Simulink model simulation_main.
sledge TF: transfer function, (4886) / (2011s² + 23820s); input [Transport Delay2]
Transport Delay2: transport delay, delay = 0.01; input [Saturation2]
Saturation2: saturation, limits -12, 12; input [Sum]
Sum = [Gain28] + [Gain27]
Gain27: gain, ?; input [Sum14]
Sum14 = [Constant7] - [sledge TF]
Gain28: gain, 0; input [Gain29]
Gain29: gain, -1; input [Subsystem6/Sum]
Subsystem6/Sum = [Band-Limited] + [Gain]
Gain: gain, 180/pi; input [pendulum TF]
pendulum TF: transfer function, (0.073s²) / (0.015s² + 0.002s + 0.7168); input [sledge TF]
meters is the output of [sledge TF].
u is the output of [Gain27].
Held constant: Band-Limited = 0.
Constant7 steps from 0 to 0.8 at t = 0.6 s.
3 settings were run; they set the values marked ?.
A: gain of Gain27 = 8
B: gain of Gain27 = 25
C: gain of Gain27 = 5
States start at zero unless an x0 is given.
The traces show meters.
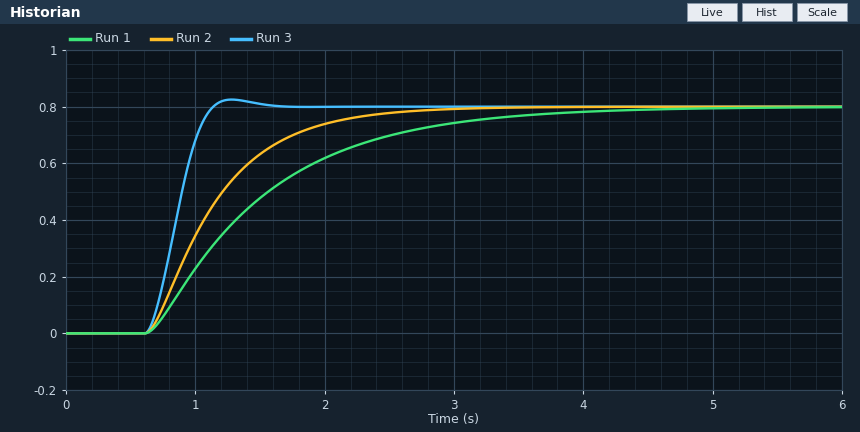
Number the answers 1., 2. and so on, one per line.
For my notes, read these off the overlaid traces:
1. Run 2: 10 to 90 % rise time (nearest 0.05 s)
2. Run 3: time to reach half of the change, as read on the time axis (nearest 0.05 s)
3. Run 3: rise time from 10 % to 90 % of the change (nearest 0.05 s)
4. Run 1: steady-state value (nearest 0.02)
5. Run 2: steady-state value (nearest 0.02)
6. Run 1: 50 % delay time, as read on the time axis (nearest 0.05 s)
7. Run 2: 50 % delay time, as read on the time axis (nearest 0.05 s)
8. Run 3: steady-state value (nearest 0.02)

1. 1.15 s
2. 0.85 s
3. 0.35 s
4. 0.80
5. 0.80
6. 1.30 s
7. 1.05 s
8. 0.80
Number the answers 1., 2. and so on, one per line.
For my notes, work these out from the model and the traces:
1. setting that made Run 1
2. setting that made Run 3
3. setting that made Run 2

1. C
2. B
3. A
